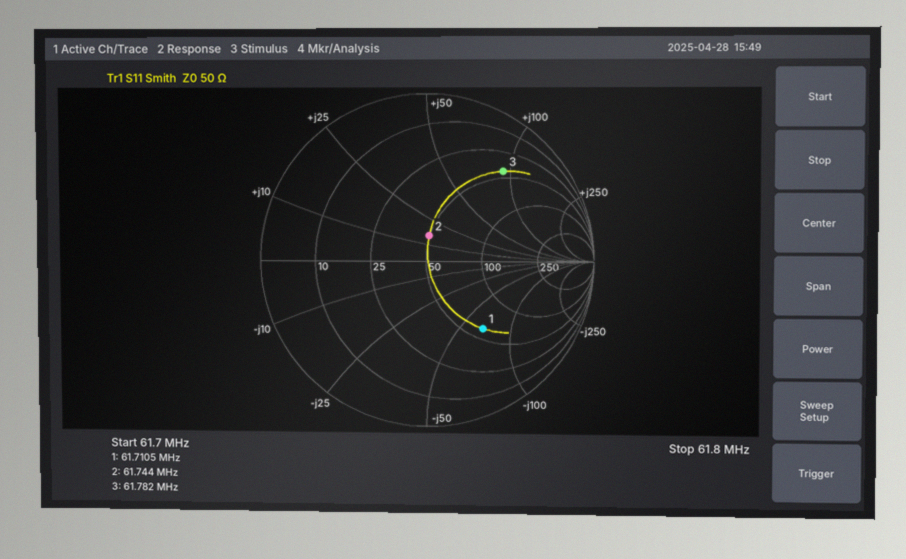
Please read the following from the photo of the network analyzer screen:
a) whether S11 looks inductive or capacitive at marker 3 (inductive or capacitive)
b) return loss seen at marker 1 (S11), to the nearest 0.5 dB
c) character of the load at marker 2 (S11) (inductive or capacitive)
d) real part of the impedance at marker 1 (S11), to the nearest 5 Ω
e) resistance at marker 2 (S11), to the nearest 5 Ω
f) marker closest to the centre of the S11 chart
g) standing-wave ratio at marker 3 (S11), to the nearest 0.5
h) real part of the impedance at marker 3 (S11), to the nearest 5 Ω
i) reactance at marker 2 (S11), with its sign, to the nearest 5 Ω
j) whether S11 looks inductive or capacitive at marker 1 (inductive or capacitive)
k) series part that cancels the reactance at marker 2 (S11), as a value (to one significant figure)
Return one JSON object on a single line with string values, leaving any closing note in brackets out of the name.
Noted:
{"whether S11 looks inductive or capacitive at marker 3": "inductive", "return loss seen at marker 1 (S11), to the nearest 0.5 dB": "5.5 dB", "character of the load at marker 2 (S11)": "inductive", "real part of the impedance at marker 1 (S11), to the nearest 5 Ω": "60 Ω", "resistance at marker 2 (S11), to the nearest 5 Ω": "50 Ω", "marker closest to the centre of the S11 chart": "marker 2", "standing-wave ratio at marker 3 (S11), to the nearest 0.5": "6.0", "real part of the impedance at marker 3 (S11), to the nearest 5 Ω": "45 Ω", "reactance at marker 2 (S11), with its sign, to the nearest 5 Ω": "+15 Ω", "whether S11 looks inductive or capacitive at marker 1": "capacitive", "series part that cancels the reactance at marker 2 (S11), as a value": "200 pF"}
